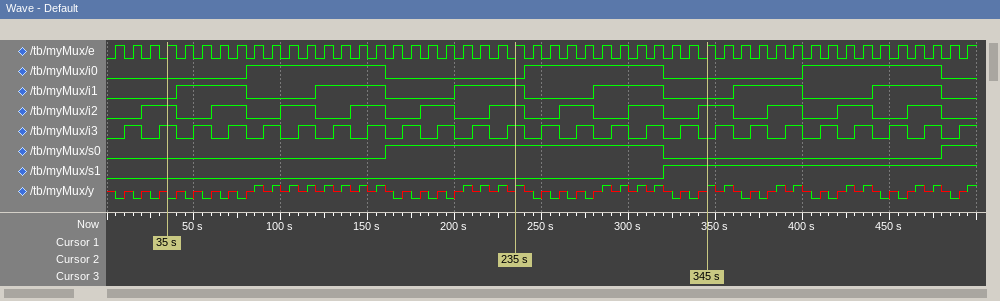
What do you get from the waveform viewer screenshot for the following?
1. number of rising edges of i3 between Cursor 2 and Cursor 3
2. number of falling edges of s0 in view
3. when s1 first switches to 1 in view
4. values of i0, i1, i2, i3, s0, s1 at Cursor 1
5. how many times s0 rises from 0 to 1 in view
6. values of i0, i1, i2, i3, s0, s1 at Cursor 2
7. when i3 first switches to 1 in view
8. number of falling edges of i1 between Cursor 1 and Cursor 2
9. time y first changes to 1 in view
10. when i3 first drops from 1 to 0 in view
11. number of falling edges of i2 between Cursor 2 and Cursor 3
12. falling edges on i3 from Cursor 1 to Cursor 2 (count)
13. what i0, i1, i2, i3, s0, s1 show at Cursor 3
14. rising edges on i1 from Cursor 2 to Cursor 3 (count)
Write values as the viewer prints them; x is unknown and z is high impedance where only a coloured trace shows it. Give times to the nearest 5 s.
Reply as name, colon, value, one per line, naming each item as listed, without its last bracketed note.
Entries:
number of rising edges of i3 between Cursor 2 and Cursor 3: 5
number of falling edges of s0 in view: 1
when s1 first switches to 1 in view: 320 s
values of i0, i1, i2, i3, s0, s1 at Cursor 1: i0=0, i1=0, i2=1, i3=1, s0=0, s1=0
how many times s0 rises from 0 to 1 in view: 2
values of i0, i1, i2, i3, s0, s1 at Cursor 2: i0=0, i1=1, i2=1, i3=1, s0=1, s1=0
when i3 first switches to 1 in view: 10 s
number of falling edges of i1 between Cursor 1 and Cursor 2: 2
time y first changes to 1 in view: 85 s
when i3 first drops from 1 to 0 in view: 20 s
number of falling edges of i2 between Cursor 2 and Cursor 3: 3
falling edges on i3 from Cursor 1 to Cursor 2: 10
what i0, i1, i2, i3, s0, s1 show at Cursor 3: i0=0, i1=0, i2=1, i3=0, s0=0, s1=1
rising edges on i1 from Cursor 2 to Cursor 3: 1
